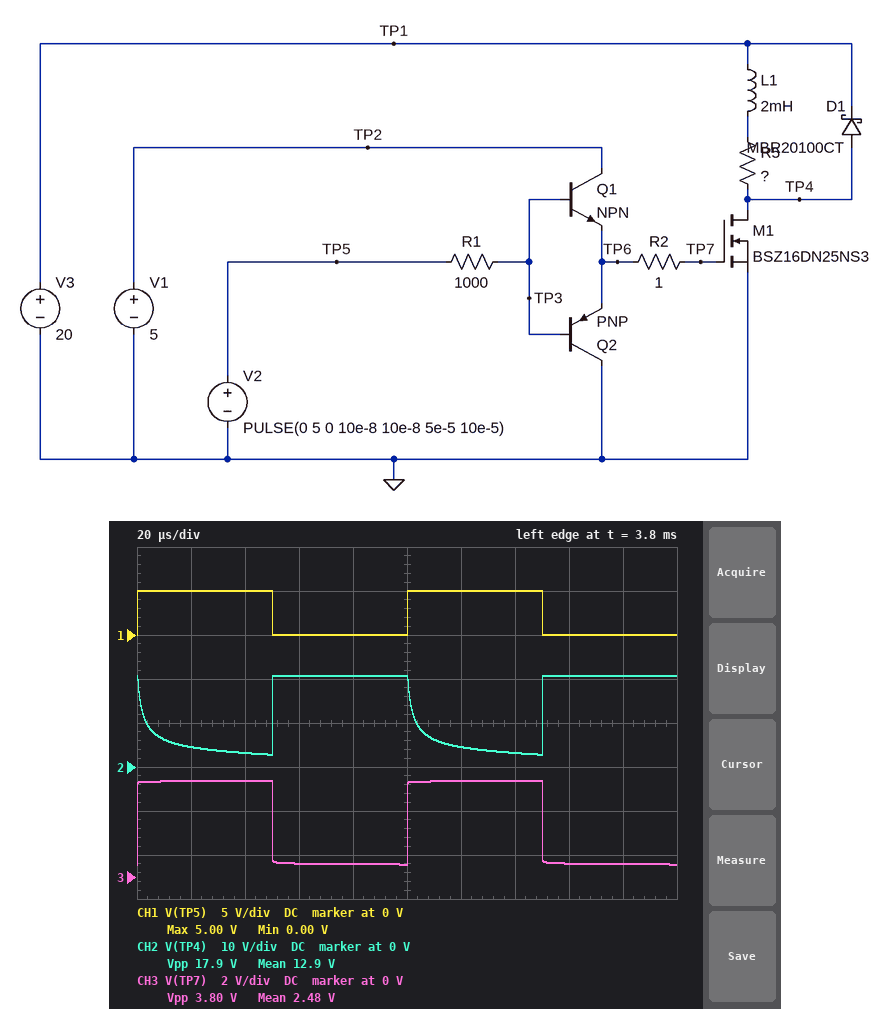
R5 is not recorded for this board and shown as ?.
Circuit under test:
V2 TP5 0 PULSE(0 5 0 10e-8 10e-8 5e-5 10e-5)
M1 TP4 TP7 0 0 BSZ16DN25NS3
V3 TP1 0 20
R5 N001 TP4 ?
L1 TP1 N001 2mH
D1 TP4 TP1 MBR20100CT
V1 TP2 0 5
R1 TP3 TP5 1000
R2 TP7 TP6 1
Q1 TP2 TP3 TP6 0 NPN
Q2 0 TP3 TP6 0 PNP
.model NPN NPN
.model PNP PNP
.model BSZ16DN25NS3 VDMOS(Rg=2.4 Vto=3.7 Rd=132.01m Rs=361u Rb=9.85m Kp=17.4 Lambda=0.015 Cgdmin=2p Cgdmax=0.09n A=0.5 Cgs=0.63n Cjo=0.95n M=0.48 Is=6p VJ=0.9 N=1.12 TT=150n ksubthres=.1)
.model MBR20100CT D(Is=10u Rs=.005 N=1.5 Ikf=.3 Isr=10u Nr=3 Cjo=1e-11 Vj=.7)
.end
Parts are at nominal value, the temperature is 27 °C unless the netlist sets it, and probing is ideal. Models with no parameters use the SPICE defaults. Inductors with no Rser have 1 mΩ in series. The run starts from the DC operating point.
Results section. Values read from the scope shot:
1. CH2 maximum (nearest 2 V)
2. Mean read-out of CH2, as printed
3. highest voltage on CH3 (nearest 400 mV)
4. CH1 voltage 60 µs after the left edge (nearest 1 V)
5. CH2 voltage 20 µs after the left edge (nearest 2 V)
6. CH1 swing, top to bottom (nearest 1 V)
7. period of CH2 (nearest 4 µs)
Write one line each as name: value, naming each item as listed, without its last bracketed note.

CH2 maximum: 20 V
Mean read-out of CH2, as printed: 12.9 V
highest voltage on CH3: 4.4 V
CH1 voltage 60 µs after the left edge: 0 V
CH2 voltage 20 µs after the left edge: 4 V
CH1 swing, top to bottom: 5 V
period of CH2: 100 µs
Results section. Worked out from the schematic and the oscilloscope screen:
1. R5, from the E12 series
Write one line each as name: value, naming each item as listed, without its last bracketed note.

R5, from the E12 series: 1.8 Ω
